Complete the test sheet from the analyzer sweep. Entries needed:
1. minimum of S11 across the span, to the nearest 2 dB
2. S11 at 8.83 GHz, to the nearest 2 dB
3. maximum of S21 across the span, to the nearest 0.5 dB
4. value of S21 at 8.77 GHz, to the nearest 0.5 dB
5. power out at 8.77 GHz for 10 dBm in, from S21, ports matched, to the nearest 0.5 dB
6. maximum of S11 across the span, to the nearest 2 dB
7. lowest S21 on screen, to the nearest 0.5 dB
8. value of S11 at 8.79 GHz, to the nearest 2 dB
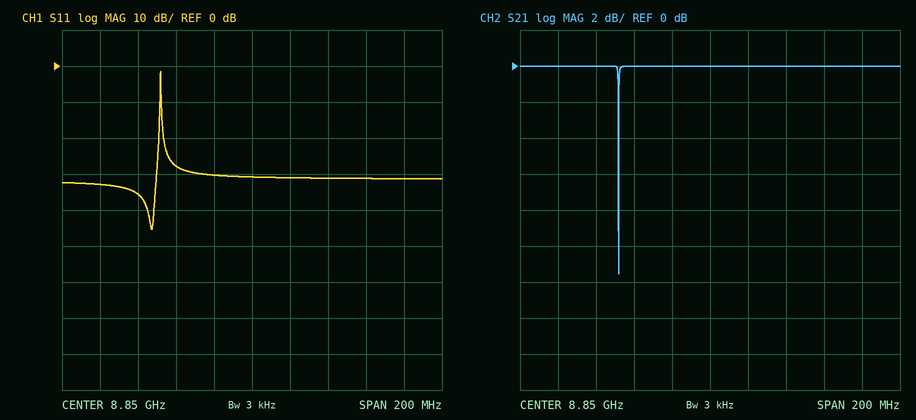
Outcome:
-46 dB
-30 dB
0.0 dB
0.0 dB
10.0 dBm
-2 dB
-11.5 dB
-36 dB
